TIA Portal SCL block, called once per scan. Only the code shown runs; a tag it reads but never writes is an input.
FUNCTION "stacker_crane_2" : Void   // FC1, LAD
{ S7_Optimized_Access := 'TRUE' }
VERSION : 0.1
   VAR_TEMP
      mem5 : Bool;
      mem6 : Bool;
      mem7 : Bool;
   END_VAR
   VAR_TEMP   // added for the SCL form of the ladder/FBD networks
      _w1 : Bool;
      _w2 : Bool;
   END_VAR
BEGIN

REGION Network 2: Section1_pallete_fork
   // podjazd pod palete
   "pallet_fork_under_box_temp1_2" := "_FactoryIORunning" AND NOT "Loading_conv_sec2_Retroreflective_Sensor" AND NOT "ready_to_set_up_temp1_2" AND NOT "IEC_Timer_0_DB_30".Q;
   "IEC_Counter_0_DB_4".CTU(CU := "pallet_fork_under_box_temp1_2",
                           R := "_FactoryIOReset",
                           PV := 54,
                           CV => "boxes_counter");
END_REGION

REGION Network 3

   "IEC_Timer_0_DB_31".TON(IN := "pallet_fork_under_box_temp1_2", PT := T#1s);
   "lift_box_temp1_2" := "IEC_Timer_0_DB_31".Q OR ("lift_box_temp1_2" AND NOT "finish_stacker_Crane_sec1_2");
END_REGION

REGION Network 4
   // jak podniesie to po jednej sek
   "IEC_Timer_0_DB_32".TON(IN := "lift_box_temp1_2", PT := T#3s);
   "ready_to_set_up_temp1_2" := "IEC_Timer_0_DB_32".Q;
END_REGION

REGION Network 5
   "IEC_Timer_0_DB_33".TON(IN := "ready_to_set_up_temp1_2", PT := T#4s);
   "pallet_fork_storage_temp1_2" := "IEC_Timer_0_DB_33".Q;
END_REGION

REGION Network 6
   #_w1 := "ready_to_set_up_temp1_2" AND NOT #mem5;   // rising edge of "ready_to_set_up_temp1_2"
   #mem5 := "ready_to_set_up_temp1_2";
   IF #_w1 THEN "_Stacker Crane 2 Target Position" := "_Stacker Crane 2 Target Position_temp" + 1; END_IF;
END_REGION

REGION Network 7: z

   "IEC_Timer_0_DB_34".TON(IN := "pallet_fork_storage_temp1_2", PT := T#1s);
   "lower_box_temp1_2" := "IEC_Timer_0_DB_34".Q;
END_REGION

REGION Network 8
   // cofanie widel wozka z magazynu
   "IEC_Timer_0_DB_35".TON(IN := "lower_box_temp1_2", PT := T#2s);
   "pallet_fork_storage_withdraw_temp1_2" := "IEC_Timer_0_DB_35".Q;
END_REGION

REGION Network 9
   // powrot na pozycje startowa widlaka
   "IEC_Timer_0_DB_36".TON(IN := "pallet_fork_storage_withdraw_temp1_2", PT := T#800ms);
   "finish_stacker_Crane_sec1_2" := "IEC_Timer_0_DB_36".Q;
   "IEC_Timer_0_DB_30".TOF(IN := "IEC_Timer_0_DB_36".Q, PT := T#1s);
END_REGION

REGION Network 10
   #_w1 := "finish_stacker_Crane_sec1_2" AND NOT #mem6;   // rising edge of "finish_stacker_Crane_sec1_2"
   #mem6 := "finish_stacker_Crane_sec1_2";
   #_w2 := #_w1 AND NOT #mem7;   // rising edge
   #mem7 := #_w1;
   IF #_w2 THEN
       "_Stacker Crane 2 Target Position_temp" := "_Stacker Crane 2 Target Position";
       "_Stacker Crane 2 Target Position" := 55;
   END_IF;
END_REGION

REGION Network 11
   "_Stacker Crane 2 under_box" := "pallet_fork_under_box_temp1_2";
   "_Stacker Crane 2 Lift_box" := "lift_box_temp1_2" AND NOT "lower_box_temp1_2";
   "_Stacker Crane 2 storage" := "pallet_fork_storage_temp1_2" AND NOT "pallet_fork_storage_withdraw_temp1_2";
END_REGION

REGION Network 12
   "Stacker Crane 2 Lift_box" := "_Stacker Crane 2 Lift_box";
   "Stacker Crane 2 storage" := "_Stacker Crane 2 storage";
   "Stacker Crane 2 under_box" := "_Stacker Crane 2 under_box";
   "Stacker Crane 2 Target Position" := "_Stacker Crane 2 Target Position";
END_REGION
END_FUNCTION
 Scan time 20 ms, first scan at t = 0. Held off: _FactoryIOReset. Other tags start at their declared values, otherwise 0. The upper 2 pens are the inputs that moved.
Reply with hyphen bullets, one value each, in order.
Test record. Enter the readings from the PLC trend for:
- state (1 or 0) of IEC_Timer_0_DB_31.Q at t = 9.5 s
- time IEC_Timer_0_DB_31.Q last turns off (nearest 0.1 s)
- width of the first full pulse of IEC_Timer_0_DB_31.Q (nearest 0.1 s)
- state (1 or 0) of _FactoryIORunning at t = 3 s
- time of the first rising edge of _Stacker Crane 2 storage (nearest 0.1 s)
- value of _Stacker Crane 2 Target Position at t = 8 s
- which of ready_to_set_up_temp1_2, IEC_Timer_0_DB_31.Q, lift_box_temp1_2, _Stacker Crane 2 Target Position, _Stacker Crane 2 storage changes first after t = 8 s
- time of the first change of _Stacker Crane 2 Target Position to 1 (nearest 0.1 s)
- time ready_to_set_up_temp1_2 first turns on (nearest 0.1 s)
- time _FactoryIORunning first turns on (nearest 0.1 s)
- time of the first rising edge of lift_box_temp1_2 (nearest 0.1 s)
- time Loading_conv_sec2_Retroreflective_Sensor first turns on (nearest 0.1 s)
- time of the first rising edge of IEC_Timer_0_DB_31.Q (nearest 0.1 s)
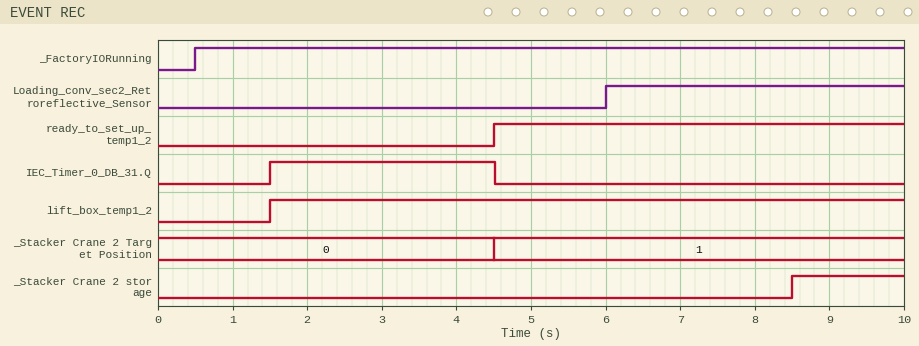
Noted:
- 0
- 4.5 s
- 3.0 s
- 1
- 8.5 s
- 1
- _Stacker Crane 2 storage
- 4.5 s
- 4.5 s
- 0.5 s
- 1.5 s
- 6.0 s
- 1.5 s
